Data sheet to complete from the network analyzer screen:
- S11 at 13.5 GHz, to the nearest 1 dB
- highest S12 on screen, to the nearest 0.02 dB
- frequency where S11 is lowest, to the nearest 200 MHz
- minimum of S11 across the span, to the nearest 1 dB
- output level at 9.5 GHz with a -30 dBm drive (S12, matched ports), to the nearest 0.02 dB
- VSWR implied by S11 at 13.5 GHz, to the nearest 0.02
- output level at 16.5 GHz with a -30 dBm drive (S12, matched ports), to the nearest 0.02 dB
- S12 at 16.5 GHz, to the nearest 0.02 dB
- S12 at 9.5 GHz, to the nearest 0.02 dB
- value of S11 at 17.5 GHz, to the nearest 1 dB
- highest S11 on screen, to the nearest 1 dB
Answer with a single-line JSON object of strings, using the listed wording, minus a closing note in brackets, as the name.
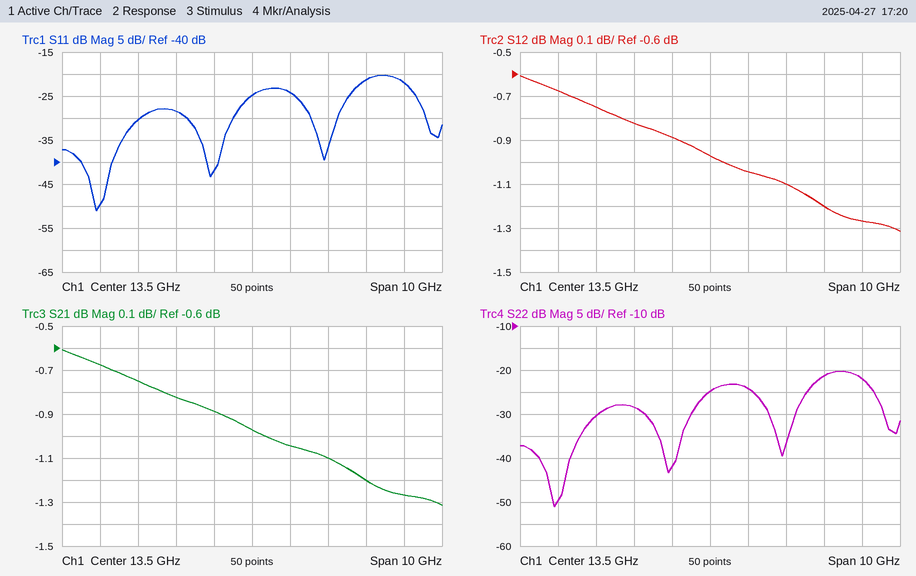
{"S11 at 13.5 GHz, to the nearest 1 dB": "-25 dB", "highest S12 on screen, to the nearest 0.02 dB": "-0.60 dB", "frequency where S11 is lowest, to the nearest 200 MHz": "9.4 GHz", "minimum of S11 across the span, to the nearest 1 dB": "-51 dB", "output level at 9.5 GHz with a -30 dBm drive (S12, matched ports), to the nearest 0.02 dB": "-30.68 dBm", "VSWR implied by S11 at 13.5 GHz, to the nearest 0.02": "1.12", "output level at 16.5 GHz with a -30 dBm drive (S12, matched ports), to the nearest 0.02 dB": "-31.20 dBm", "S12 at 16.5 GHz, to the nearest 0.02 dB": "-1.20 dB", "S12 at 9.5 GHz, to the nearest 0.02 dB": "-0.68 dB", "value of S11 at 17.5 GHz, to the nearest 1 dB": "-22 dB", "highest S11 on screen, to the nearest 1 dB": "-20 dB"}
